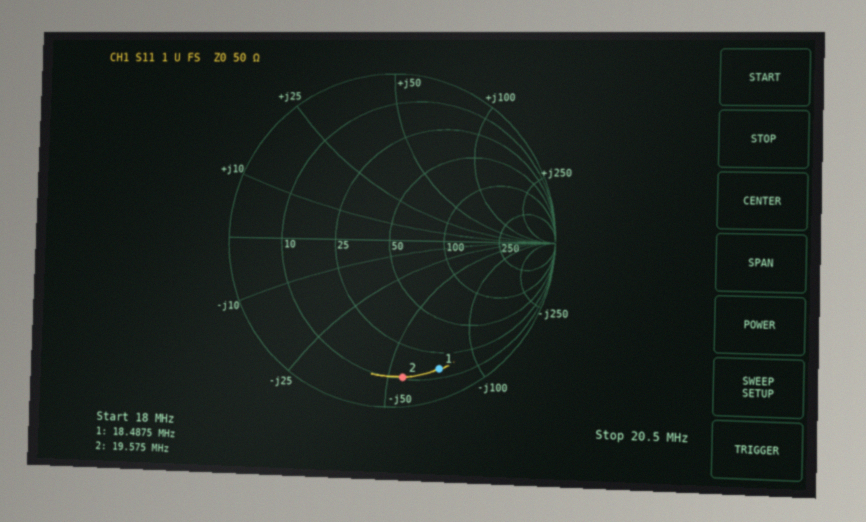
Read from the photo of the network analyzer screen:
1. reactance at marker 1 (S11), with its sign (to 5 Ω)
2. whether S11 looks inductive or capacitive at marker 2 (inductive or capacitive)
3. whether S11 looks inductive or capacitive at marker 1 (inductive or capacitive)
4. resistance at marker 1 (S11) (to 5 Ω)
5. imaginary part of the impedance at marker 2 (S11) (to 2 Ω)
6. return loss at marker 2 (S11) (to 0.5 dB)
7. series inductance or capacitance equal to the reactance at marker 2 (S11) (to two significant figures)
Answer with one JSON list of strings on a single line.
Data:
["-75 Ω", "capacitive", "capacitive", "15 Ω", "-56 Ω", "1.5 dB", "150 pF"]
